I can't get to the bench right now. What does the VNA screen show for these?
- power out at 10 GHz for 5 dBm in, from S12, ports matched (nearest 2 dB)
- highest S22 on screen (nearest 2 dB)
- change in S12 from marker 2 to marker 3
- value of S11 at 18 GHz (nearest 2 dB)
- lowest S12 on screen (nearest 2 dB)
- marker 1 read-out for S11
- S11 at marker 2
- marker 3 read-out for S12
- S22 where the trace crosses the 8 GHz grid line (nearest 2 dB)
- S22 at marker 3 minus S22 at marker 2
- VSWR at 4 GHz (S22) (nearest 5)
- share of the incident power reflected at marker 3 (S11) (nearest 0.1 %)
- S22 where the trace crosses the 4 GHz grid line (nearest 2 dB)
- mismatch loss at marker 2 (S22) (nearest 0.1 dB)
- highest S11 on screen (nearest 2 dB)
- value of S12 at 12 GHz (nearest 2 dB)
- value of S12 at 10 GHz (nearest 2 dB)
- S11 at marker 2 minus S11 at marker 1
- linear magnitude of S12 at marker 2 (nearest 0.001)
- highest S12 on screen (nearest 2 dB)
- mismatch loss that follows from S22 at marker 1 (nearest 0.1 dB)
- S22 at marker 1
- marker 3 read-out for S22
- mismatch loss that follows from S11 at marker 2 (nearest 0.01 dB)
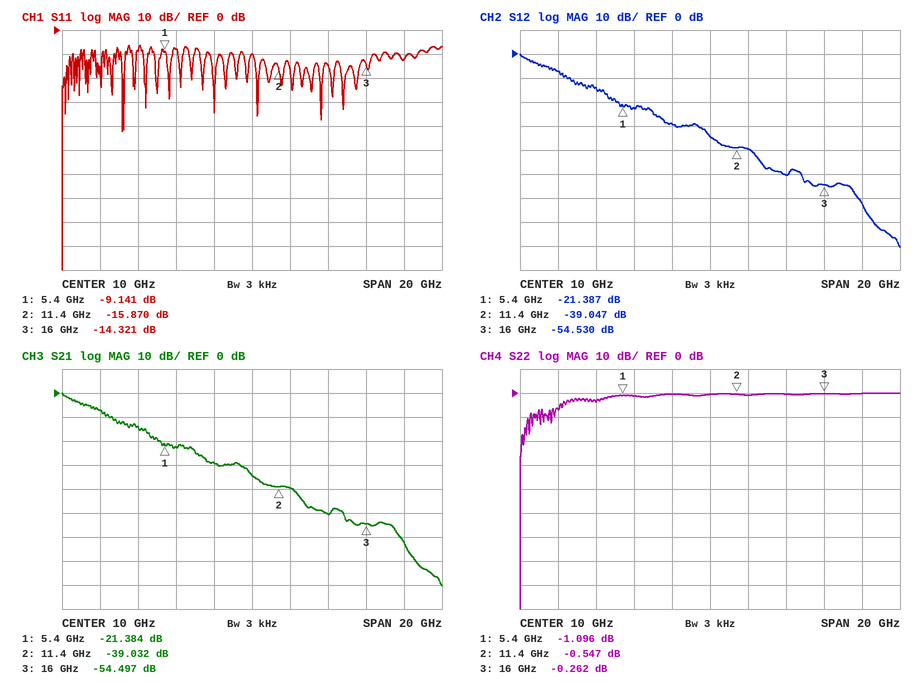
-30 dBm
0 dB
-15.483 dB
-12 dB
-80 dB
-9.141 dB
-15.870 dB
-54.530 dB
0 dB
0.285 dB
5
3.7 %
-4 dB
9.3 dB
-6 dB
-40 dB
-34 dB
-6.729 dB
0.011
0 dB
6.5 dB
-1.096 dB
-0.262 dB
0.11 dB
